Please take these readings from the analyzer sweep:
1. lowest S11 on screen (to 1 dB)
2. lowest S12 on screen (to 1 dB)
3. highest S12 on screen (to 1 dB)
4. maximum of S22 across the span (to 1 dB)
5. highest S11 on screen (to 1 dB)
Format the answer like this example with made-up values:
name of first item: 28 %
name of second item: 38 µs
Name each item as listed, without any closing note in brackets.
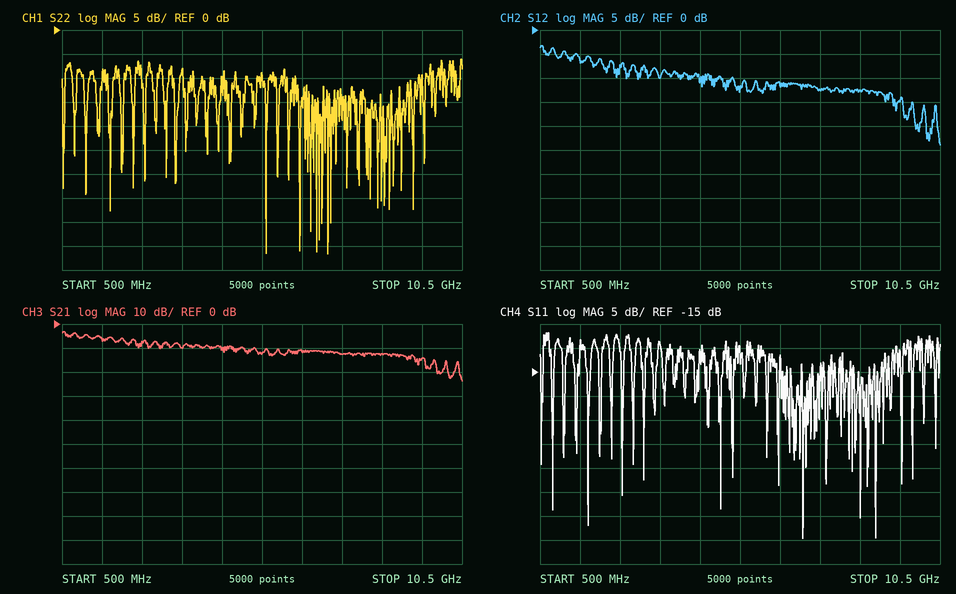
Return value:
lowest S11 on screen: -50 dB
lowest S12 on screen: -24 dB
highest S12 on screen: -3 dB
maximum of S22 across the span: -6 dB
highest S11 on screen: -7 dB
